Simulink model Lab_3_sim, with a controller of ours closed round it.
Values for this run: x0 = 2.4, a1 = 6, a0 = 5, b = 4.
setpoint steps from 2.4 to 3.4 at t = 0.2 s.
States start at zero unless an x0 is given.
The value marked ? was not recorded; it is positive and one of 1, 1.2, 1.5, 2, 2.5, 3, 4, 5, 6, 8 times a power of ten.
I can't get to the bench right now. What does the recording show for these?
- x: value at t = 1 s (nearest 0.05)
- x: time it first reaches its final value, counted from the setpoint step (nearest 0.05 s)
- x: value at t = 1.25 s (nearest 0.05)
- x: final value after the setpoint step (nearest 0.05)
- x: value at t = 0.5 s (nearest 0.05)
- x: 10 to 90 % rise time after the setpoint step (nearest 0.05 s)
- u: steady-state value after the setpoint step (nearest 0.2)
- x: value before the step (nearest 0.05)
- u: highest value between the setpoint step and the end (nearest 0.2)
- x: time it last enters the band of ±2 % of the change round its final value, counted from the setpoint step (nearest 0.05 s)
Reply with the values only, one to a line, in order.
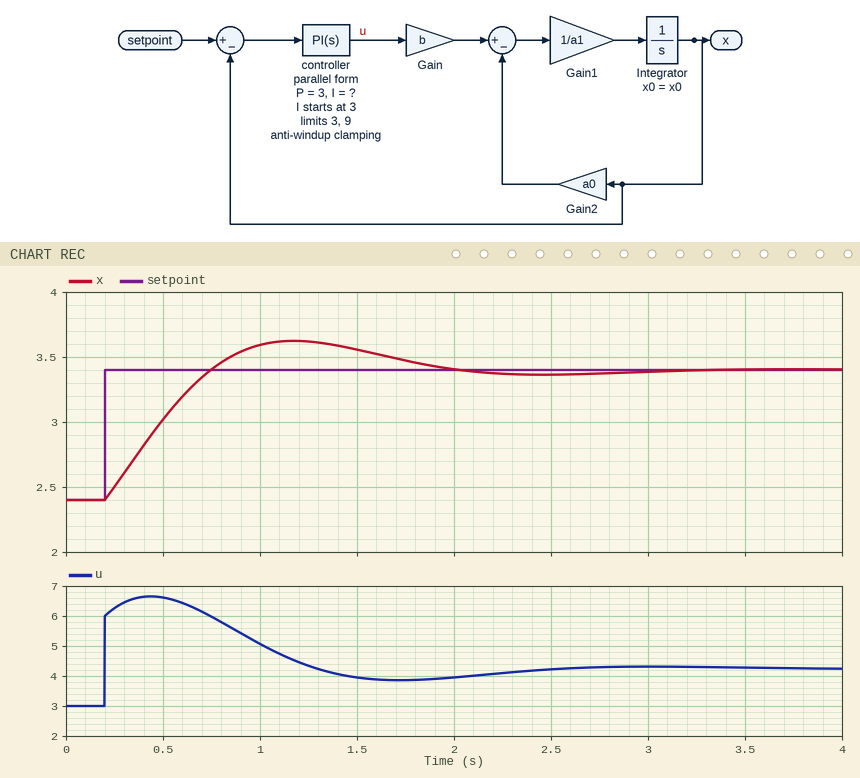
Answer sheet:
3.60
0.55 s
3.60
3.40
3.00
0.40 s
4.2
2.40
6.6
2.70 s
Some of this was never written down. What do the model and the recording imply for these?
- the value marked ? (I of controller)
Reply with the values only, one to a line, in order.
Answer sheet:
12
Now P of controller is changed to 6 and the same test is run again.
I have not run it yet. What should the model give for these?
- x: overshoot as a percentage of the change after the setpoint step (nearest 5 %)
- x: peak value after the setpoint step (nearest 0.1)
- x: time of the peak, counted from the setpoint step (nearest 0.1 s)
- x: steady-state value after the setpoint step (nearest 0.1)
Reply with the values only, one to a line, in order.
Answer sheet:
10 %
3.5
0.9 s
3.4
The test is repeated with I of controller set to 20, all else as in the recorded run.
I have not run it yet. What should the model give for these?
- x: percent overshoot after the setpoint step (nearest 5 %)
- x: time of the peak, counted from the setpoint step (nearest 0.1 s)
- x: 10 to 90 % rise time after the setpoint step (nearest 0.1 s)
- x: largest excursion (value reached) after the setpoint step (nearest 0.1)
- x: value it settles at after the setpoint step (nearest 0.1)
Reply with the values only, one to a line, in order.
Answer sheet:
30 %
0.8 s
0.3 s
3.7
3.4
